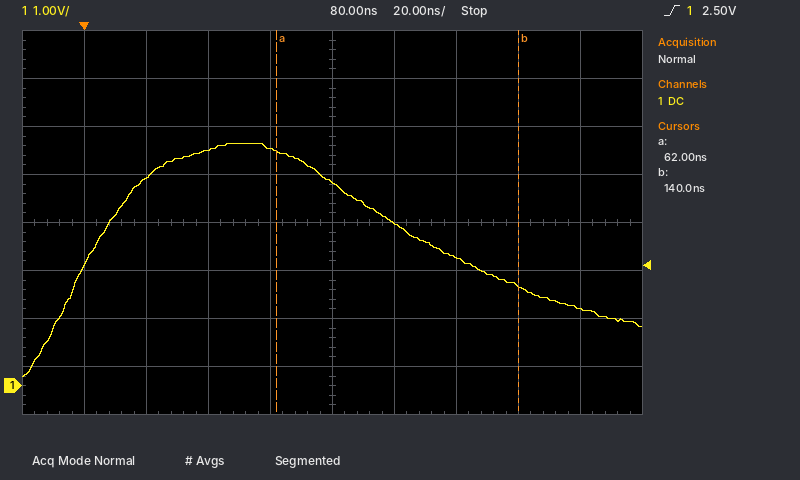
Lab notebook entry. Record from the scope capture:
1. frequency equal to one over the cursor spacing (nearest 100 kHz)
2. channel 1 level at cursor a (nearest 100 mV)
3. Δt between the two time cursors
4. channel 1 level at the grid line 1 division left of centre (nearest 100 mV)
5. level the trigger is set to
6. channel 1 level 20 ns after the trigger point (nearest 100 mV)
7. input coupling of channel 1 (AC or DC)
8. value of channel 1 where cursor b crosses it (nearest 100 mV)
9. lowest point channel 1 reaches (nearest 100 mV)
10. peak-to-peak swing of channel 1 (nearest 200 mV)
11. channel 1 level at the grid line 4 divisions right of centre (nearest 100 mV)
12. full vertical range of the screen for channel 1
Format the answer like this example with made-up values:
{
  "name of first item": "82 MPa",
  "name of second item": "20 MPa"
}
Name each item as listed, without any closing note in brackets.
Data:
{
  "frequency equal to one over the cursor spacing": "12.8 MHz",
  "channel 1 level at cursor a": "4.9 V",
  "Δt between the two time cursors": "78 ns",
  "channel 1 level at the grid line 1 division left of centre": "4.9 V",
  "level the trigger is set to": "2.50 V",
  "channel 1 level 20 ns after the trigger point": "4.3 V",
  "input coupling of channel 1": "DC",
  "value of channel 1 where cursor b crosses it": "2.1 V",
  "lowest point channel 1 reaches": "200 mV",
  "peak-to-peak swing of channel 1": "4.8 V",
  "channel 1 level at the grid line 4 divisions right of centre": "1.6 V",
  "full vertical range of the screen for channel 1": "8 V"
}
